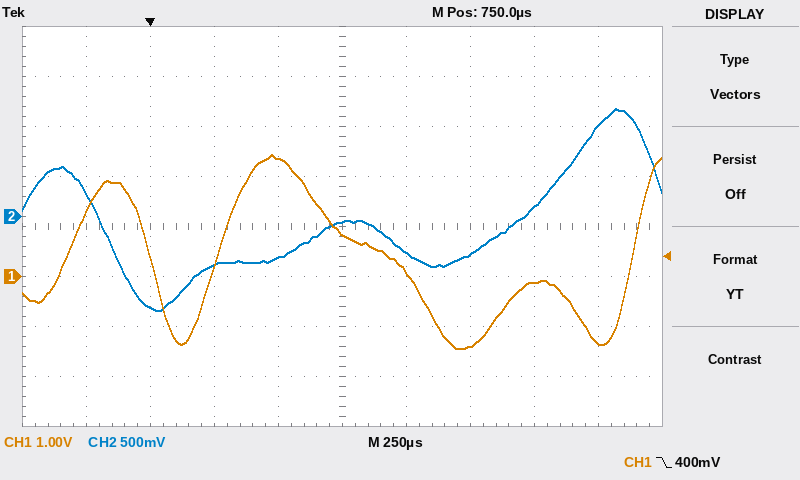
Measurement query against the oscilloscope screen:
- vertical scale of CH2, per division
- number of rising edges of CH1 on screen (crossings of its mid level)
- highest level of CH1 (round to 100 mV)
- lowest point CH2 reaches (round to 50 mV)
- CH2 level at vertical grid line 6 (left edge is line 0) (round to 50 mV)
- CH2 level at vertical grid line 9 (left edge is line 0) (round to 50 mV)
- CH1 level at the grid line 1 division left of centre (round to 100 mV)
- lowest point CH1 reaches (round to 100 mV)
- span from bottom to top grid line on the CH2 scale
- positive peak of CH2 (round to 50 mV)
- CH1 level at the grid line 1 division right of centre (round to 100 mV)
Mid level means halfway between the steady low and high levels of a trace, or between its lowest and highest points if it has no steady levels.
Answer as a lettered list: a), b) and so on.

a) 500 mV
b) 3
c) 2.4 V
d) -950 mV
e) -350 mV
f) 900 mV
g) 2.4 V
h) -1.4 V
i) 4 V
j) 1.10 V
k) 100 mV
